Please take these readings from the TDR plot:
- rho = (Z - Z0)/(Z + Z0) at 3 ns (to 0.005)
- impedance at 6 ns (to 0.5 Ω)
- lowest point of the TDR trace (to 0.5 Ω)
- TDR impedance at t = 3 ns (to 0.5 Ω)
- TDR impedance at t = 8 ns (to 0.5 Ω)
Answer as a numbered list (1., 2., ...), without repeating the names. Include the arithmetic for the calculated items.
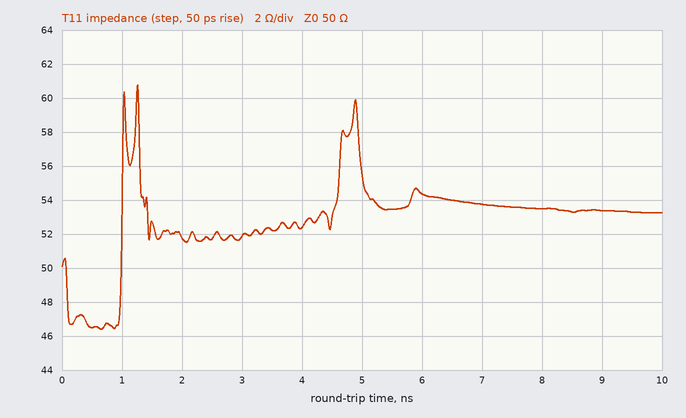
1. (52 − 50)/(52 + 50) ≈ +0.020
2. 54.5 Ω
3. 46.5 Ω
4. 52.0 Ω
5. 53.5 Ω
